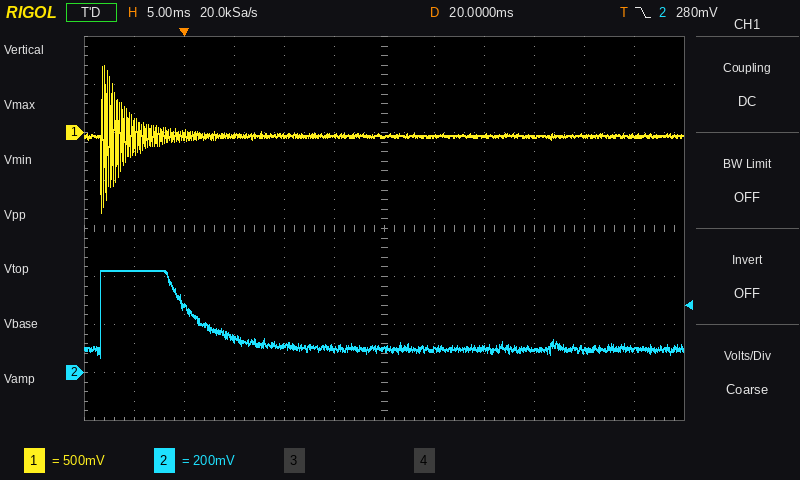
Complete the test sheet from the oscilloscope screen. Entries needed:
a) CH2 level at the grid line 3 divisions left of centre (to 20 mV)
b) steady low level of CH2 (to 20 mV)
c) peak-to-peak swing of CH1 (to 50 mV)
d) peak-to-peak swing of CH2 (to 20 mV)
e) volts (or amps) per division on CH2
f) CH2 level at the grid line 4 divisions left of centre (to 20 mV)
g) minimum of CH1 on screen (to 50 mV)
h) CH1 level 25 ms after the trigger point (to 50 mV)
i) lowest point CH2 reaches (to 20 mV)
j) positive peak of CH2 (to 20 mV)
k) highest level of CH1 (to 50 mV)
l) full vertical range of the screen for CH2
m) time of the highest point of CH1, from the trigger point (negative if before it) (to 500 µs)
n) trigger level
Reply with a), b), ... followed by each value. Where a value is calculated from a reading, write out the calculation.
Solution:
a) 140 mV
b) 100 mV
c) 700 mV − (-850 mV) = 1.55 V
d) 420 mV − (60 mV) = 360 mV
e) 200 mV
f) 280 mV
g) -850 mV
h) -50 mV
i) 60 mV
j) 420 mV
k) 700 mV
l) 1.6 V
m) -8.0 ms
n) 280 mV
